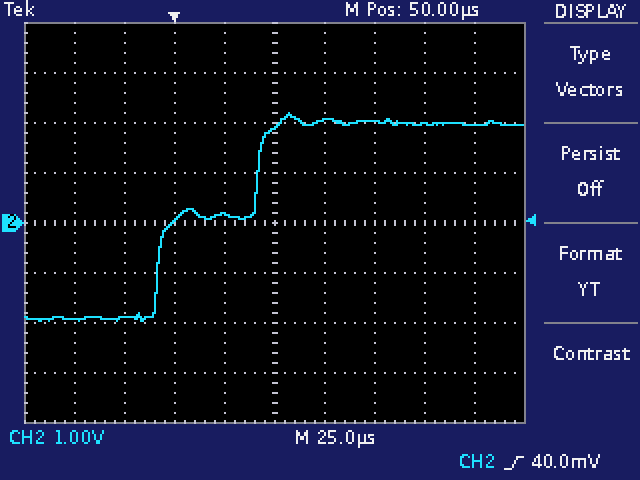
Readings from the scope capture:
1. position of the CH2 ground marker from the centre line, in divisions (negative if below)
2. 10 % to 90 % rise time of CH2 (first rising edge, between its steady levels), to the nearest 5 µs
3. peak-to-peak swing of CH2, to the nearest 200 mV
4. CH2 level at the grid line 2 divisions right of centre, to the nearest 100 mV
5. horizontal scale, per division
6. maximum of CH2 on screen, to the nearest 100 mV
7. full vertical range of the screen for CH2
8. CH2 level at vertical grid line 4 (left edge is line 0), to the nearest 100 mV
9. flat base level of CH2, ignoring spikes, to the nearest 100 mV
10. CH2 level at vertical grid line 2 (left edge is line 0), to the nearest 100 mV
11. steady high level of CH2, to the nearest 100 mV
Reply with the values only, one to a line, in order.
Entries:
0.0 div
55 µs
4.2 V
2.0 V
25 µs
2.2 V
8 V
200 mV
-1.9 V
-1.9 V
2.0 V
